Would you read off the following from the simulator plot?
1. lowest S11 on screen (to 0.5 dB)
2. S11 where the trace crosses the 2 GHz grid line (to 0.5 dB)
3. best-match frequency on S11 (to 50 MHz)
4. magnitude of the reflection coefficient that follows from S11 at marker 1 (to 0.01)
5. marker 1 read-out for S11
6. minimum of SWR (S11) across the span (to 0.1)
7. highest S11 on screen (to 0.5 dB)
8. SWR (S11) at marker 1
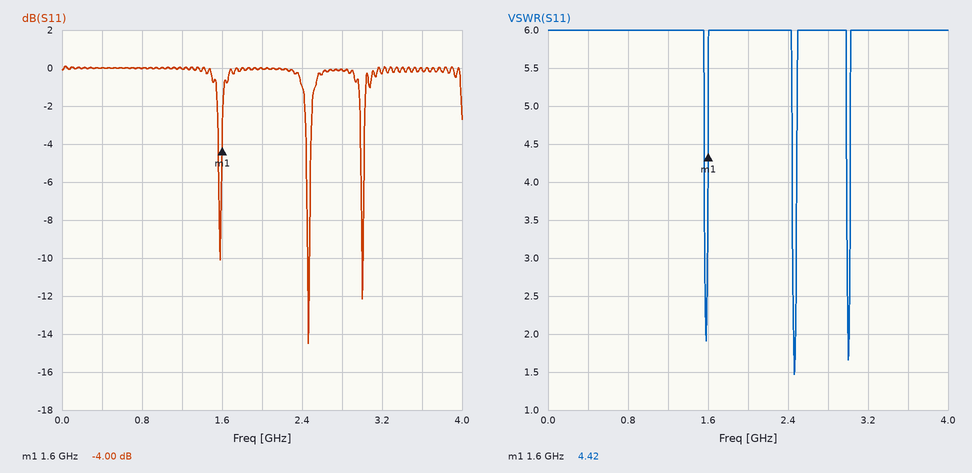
-14.5 dB
0.0 dB
2.45 GHz
0.63
-4.00 dB
1.5
0.0 dB
4.42
